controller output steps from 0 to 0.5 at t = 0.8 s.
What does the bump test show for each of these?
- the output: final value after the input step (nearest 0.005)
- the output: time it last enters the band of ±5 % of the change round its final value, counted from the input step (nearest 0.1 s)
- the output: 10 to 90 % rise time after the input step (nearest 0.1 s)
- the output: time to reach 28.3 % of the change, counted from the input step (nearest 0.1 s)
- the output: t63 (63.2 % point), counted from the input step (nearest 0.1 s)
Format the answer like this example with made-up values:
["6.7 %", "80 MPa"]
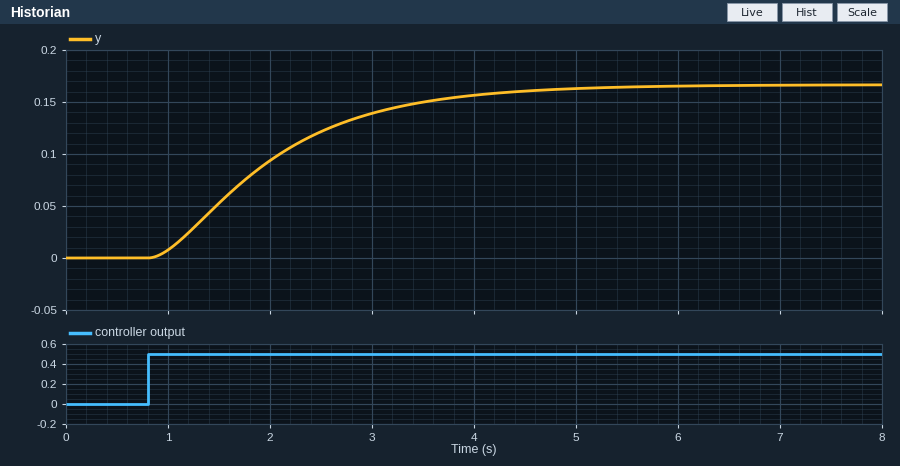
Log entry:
["0.165", "3.4 s", "2.4 s", "0.6 s", "1.4 s"]
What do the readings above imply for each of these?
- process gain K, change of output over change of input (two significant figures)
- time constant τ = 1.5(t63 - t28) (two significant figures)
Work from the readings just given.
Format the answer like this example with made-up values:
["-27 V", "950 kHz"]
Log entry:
["0.33", "1.2 s"]
